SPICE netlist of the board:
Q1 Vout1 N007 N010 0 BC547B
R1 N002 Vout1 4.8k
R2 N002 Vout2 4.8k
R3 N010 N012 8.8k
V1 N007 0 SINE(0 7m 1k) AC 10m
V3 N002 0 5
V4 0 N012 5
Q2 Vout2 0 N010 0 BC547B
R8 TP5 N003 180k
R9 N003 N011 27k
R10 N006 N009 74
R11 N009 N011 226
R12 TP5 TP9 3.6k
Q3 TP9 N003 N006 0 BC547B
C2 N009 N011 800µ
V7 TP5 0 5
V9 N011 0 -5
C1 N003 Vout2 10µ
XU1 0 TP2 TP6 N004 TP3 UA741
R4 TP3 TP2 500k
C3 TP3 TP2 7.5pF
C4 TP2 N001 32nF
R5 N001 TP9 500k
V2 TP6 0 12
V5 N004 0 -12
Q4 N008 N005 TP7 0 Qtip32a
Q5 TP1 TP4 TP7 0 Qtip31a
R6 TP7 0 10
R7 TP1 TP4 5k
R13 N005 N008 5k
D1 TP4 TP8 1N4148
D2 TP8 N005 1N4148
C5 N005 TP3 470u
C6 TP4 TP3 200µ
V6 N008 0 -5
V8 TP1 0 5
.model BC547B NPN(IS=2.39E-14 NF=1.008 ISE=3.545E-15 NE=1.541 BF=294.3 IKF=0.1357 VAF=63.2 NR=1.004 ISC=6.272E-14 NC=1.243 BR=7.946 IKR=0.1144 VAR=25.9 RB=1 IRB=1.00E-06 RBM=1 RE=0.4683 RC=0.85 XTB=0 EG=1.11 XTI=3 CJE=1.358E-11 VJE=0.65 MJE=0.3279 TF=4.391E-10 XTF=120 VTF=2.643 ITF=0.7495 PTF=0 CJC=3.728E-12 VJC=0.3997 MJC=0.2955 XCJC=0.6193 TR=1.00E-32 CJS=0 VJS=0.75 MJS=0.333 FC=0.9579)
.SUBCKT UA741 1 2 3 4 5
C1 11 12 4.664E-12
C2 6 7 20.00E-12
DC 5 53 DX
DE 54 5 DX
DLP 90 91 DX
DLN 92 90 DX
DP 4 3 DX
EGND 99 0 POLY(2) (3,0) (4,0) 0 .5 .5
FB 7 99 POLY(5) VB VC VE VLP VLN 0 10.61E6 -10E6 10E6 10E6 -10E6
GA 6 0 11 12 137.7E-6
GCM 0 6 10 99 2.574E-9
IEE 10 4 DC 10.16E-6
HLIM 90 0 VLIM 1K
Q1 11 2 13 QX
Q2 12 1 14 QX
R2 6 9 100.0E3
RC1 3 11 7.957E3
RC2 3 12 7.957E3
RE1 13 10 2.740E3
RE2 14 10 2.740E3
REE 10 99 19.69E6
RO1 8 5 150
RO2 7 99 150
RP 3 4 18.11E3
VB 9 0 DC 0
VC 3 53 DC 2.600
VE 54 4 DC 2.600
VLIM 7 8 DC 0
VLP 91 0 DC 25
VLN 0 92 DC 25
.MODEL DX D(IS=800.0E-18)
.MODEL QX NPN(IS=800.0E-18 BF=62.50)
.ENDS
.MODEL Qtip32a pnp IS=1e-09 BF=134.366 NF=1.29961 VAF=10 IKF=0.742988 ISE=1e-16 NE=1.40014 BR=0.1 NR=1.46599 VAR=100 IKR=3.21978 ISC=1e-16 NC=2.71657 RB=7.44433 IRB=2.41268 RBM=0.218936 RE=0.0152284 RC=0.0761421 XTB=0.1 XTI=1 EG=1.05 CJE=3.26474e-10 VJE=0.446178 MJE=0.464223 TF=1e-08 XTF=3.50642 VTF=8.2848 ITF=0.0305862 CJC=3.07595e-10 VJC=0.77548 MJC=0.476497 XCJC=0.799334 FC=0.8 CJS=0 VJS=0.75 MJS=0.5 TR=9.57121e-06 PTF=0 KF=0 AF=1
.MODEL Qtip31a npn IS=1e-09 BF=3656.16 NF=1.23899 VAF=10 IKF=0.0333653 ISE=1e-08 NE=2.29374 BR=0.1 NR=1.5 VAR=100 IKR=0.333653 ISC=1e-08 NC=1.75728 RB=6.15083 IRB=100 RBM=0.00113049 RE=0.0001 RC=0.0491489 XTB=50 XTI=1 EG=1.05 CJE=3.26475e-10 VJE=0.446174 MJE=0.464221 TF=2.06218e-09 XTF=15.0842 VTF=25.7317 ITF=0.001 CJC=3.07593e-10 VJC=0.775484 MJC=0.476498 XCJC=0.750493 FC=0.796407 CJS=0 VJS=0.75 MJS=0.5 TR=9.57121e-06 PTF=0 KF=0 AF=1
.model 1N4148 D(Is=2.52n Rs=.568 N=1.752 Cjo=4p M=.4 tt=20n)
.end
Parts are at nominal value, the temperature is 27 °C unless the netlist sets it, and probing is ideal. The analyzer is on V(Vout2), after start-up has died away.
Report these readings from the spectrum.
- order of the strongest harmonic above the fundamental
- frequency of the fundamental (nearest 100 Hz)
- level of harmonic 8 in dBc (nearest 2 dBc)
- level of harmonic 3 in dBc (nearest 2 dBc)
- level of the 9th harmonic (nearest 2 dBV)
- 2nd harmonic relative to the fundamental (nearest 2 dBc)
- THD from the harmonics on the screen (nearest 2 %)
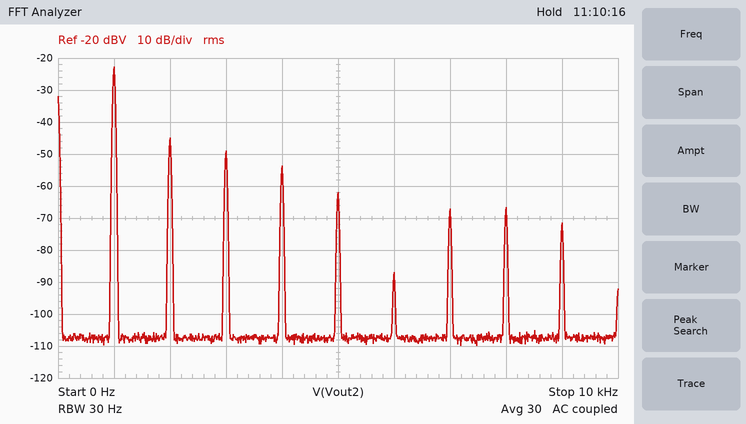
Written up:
2
1.0 kHz
-44 dBc
-26 dBc
-72 dBV
-22 dBc
10 %
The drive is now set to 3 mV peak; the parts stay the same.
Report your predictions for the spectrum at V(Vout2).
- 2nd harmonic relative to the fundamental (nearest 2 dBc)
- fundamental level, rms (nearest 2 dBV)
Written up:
-48 dBc
-30 dBV
